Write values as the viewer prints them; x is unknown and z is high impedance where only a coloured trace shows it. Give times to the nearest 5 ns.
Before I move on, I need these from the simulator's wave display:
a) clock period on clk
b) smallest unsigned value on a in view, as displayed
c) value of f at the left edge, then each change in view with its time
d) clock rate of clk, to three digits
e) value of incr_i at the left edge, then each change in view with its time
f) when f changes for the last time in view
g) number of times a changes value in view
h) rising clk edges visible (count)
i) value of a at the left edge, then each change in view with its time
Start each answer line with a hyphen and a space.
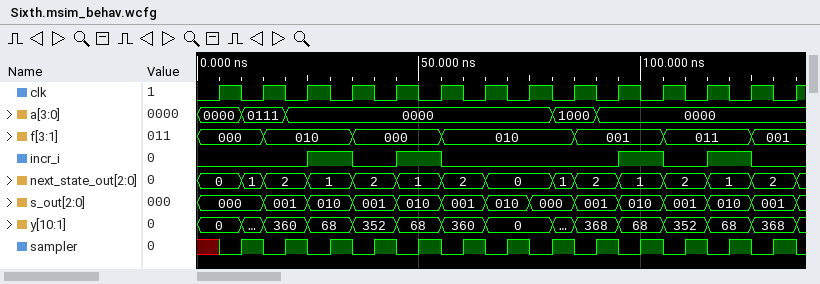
- 10 ns
- 0000
- 000, 010 at 15 ns, 000 at 35 ns, 010 at 55 ns, 001 at 85 ns, 011 at 105 ns, 001 at 125 ns
- 100 MHz
- 0, 1 at 25 ns, 0 at 35 ns, 1 at 45 ns, 0 at 55 ns, 1 at 95 ns, 0 at 105 ns, 1 at 115 ns, 0 at 125 ns
- 125 ns
- 4
- 14
- 0000, 0111 at 10 ns, 0000 at 20 ns, 1000 at 80 ns, 0000 at 90 ns
